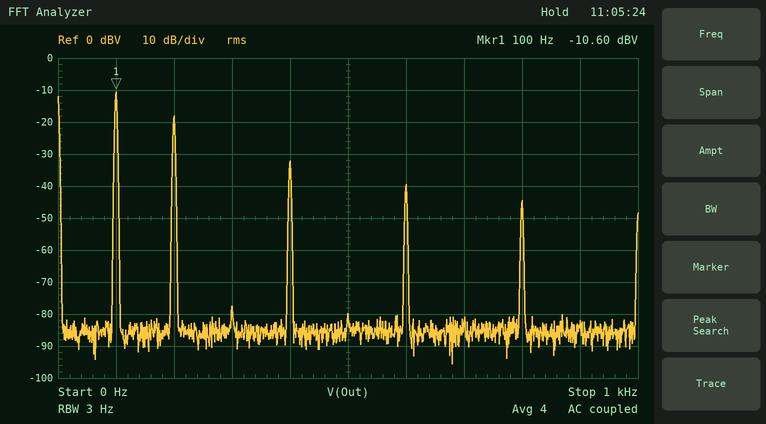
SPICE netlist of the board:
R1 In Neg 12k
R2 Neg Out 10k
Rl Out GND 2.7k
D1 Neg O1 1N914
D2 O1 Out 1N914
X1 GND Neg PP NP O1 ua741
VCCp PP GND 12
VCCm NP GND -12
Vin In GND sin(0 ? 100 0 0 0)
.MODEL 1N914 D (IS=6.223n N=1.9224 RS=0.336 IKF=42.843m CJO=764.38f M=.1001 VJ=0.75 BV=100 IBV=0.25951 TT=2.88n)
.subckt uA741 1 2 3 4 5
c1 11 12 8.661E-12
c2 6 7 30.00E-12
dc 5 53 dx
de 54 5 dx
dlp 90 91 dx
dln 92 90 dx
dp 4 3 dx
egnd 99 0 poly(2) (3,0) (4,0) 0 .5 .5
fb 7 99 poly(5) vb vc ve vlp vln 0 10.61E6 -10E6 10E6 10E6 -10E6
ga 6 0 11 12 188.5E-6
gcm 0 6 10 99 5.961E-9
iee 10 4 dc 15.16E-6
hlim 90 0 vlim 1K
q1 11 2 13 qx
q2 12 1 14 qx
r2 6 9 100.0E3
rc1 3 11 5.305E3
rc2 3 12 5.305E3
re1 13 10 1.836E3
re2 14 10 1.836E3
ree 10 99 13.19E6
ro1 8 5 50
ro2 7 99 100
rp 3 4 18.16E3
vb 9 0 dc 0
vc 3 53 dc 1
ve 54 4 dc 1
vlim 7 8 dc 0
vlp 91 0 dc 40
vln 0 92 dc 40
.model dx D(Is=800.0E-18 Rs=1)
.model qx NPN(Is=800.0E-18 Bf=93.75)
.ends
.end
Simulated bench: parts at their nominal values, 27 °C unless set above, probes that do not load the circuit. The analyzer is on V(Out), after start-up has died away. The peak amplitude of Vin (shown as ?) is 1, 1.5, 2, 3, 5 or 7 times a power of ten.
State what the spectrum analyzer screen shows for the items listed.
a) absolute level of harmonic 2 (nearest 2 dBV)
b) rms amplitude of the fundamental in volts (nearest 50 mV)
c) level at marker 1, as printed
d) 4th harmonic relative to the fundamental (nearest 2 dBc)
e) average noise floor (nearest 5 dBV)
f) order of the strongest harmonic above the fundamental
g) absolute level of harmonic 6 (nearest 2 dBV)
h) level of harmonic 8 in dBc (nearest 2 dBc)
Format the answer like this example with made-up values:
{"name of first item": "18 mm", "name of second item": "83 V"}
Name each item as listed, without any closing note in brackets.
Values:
{"absolute level of harmonic 2": "-18 dBV", "rms amplitude of the fundamental in volts": "300 mV", "level at marker 1, as printed": "-10.60 dBV", "4th harmonic relative to the fundamental": "-22 dBc", "average noise floor": "-85 dBV", "order of the strongest harmonic above the fundamental": "2", "absolute level of harmonic 6": "-40 dBV", "level of harmonic 8 in dBc": "-34 dBc"}
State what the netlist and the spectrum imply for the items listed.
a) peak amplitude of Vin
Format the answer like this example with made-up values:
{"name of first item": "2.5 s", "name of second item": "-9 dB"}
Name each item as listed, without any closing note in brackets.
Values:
{"peak amplitude of Vin": "1 V"}
